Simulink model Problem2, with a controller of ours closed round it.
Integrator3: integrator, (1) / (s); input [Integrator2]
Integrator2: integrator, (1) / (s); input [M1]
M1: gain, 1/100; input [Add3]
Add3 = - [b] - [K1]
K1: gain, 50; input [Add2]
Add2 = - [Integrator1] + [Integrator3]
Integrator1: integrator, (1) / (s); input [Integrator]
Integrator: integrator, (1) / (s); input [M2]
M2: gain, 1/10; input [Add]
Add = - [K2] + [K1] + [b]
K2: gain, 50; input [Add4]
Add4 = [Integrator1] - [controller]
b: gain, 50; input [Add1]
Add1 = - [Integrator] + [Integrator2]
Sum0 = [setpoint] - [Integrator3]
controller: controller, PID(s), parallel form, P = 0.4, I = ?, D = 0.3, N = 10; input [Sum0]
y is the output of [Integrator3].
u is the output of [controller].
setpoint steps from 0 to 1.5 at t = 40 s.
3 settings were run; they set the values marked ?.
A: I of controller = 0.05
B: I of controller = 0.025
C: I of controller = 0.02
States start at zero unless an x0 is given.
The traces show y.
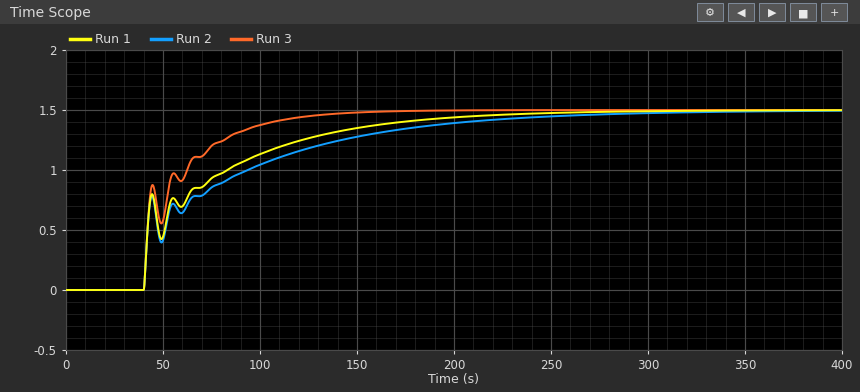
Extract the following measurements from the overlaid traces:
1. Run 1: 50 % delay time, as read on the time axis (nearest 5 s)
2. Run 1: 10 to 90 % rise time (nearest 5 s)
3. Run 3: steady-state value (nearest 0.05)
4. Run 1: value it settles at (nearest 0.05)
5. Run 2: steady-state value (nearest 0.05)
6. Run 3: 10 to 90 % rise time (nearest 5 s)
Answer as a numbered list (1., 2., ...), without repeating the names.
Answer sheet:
1. 45 s
2. 110 s
3. 1.50
4. 1.50
5. 1.50
6. 55 s
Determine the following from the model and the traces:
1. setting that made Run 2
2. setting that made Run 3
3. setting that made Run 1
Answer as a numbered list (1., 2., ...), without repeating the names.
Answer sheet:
1. C
2. A
3. B
